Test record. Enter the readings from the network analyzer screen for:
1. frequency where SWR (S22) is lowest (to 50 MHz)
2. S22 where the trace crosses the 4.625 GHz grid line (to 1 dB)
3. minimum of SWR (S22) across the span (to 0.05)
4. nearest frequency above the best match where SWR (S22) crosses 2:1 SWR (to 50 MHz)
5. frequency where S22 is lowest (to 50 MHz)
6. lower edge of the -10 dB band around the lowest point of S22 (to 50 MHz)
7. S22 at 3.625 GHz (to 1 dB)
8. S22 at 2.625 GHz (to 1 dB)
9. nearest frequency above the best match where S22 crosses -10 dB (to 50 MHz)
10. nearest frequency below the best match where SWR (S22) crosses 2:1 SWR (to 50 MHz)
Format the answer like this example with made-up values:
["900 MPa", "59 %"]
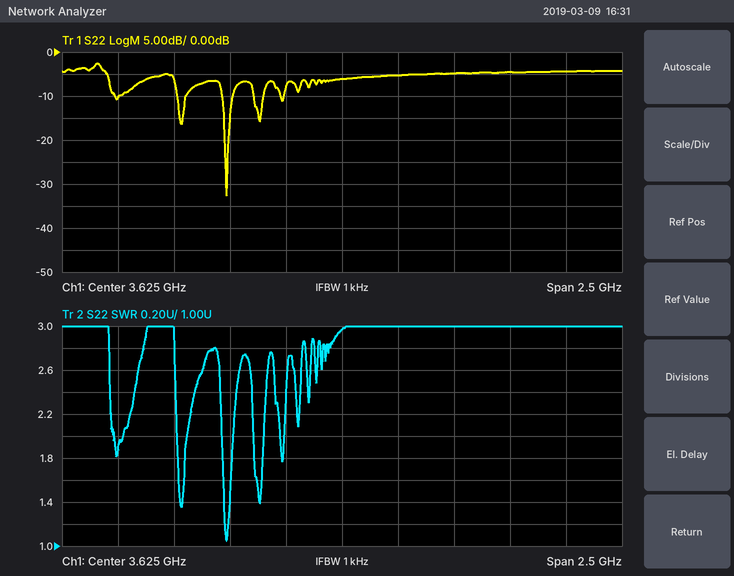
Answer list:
["3.10 GHz", "-4 dB", "1.05", "3.15 GHz", "3.10 GHz", "3.10 GHz", "-6 dB", "-10 dB", "3.15 GHz", "3.10 GHz"]
